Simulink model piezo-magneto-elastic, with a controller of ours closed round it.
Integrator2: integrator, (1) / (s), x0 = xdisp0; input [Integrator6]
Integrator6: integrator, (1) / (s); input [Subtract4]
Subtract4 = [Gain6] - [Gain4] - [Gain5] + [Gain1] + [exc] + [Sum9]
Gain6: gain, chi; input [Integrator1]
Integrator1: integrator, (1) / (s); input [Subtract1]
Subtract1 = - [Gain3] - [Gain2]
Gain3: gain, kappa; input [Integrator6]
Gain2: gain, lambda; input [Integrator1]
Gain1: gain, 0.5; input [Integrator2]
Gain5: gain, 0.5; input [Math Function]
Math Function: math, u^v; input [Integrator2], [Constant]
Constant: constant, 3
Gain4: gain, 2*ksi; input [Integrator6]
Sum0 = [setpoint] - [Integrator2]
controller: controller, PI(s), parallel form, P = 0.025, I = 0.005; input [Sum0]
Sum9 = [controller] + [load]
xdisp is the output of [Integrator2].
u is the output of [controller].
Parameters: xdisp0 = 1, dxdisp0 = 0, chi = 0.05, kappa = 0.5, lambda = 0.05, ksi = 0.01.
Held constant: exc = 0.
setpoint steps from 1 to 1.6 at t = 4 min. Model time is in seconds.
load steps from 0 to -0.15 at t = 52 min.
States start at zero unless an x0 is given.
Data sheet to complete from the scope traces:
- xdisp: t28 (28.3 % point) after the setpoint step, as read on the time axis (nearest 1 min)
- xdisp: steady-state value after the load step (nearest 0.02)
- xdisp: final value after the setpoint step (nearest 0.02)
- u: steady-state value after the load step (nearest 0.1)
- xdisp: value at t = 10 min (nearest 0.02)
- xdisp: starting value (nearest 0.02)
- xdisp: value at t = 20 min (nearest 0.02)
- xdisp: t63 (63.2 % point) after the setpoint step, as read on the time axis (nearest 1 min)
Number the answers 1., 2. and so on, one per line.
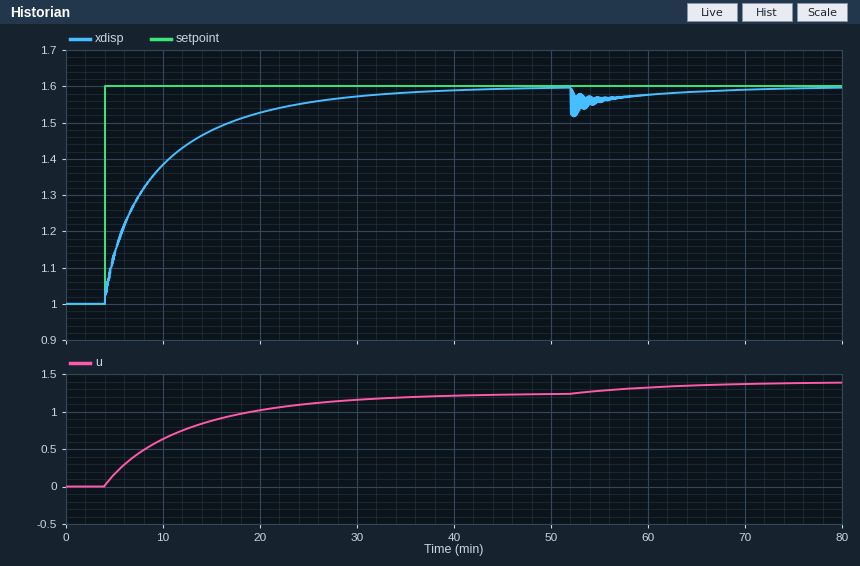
1. 5 min
2. 1.60
3. 1.60
4. 1.4
5. 1.38
6. 1.00
7. 1.52
8. 10 min
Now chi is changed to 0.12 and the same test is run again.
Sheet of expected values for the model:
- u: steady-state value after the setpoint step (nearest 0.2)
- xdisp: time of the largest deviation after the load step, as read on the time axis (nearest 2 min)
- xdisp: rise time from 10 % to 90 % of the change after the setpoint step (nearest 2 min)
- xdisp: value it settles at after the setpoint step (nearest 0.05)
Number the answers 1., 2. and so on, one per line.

1. 1.2
2. 52 min
3. 18 min
4. 1.60
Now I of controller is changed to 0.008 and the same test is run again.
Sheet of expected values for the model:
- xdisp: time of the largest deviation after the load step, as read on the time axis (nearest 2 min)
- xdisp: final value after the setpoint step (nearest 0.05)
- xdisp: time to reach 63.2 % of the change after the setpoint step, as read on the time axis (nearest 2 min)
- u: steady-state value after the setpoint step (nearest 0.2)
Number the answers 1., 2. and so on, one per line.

1. 52 min
2. 1.60
3. 8 min
4. 1.2
